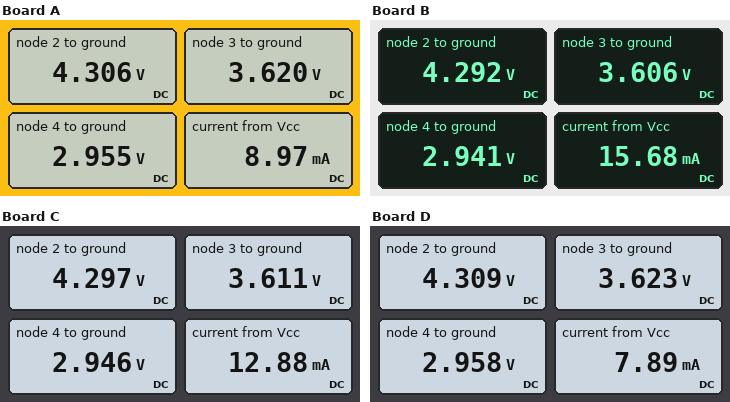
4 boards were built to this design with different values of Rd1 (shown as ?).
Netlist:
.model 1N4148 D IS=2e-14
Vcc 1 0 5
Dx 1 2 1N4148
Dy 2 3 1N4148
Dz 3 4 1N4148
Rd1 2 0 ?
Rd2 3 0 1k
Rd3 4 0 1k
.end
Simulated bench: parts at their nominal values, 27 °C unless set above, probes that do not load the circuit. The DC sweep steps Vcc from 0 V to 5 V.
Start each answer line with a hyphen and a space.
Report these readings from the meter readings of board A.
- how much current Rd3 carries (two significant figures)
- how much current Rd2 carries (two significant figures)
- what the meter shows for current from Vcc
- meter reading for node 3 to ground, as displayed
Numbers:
- 3.0 mA
- 3.6 mA
- 8.97 mA
- 3.620 V
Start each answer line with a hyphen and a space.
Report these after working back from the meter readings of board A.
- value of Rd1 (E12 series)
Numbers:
- 1.8 kΩ
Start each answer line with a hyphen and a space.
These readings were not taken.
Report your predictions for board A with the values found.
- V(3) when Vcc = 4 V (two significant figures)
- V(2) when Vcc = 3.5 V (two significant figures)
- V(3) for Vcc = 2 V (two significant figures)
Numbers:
- 2.6 V
- 2.8 V
- 720 mV
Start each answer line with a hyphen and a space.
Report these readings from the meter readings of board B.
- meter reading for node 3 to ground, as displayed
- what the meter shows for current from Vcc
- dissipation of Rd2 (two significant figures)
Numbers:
- 3.606 V
- 15.68 mA
- 13 mW
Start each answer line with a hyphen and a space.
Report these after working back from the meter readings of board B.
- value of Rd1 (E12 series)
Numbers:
- 470 Ω
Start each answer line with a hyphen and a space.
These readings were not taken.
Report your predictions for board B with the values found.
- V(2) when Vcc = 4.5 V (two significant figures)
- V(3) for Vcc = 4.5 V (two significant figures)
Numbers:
- 3.8 V
- 3.1 V
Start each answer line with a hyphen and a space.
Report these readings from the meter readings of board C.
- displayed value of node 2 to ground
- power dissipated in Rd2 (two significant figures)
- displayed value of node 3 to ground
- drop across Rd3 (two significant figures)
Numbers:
- 4.297 V
- 13 mW
- 3.611 V
- 2.9 V
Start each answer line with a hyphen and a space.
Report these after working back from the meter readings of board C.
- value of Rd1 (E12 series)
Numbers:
- 680 Ω
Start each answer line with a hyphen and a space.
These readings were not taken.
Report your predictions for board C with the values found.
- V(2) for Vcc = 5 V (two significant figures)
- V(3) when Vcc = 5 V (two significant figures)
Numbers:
- 4.3 V
- 3.6 V
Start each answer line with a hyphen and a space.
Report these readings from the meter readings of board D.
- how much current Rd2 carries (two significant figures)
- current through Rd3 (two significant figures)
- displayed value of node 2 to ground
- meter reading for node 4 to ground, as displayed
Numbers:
- 3.6 mA
- 3.0 mA
- 4.309 V
- 2.958 V
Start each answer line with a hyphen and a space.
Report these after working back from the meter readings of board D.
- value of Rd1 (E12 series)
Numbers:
- 3.3 kΩ
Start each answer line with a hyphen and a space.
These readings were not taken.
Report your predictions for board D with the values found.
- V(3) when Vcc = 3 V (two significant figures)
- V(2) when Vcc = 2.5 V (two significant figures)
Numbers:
- 1.7 V
- 1.8 V
